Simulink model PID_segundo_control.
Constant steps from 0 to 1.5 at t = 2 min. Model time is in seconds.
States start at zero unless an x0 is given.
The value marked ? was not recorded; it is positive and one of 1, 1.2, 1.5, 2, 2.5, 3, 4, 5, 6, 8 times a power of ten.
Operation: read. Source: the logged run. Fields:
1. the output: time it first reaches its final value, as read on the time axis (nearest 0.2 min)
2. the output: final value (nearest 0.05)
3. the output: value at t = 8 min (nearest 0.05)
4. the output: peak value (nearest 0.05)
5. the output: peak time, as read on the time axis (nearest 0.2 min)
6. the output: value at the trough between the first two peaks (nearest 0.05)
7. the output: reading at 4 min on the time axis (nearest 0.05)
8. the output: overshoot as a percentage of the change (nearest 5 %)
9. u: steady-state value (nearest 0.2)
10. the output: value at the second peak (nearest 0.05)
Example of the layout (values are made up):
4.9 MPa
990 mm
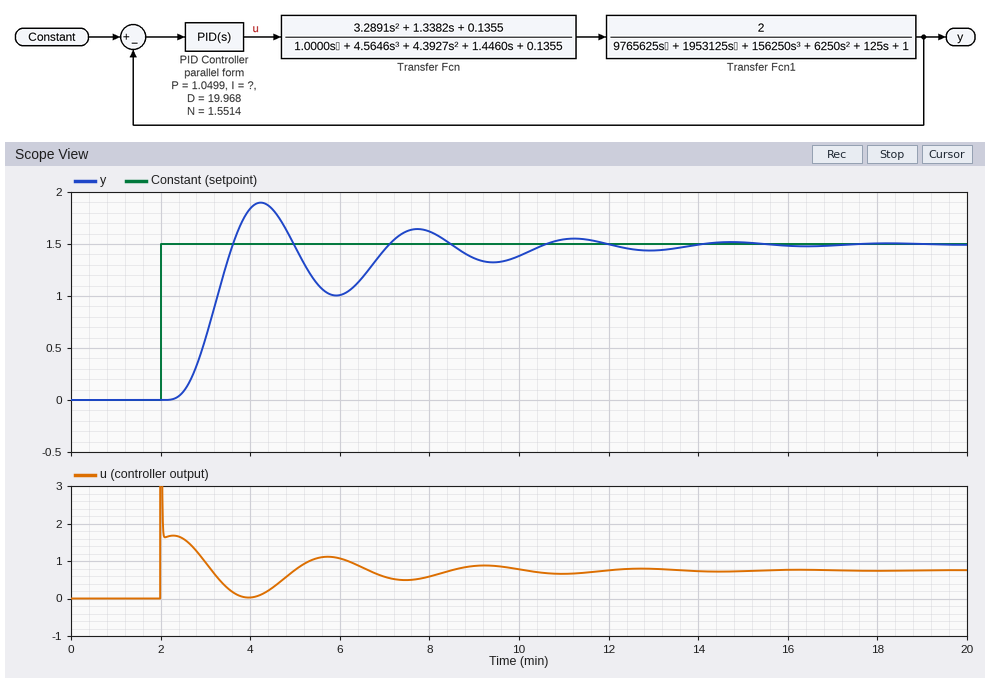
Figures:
3.6 min
1.50
1.60
1.90
4.2 min
1.00
1.85
25 %
0.8
1.65
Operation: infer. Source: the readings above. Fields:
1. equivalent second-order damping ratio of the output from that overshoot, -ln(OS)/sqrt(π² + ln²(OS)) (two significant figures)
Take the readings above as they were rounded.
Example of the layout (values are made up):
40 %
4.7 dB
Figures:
0.40
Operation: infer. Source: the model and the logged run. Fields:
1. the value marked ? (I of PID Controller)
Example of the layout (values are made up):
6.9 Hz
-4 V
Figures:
0.006
